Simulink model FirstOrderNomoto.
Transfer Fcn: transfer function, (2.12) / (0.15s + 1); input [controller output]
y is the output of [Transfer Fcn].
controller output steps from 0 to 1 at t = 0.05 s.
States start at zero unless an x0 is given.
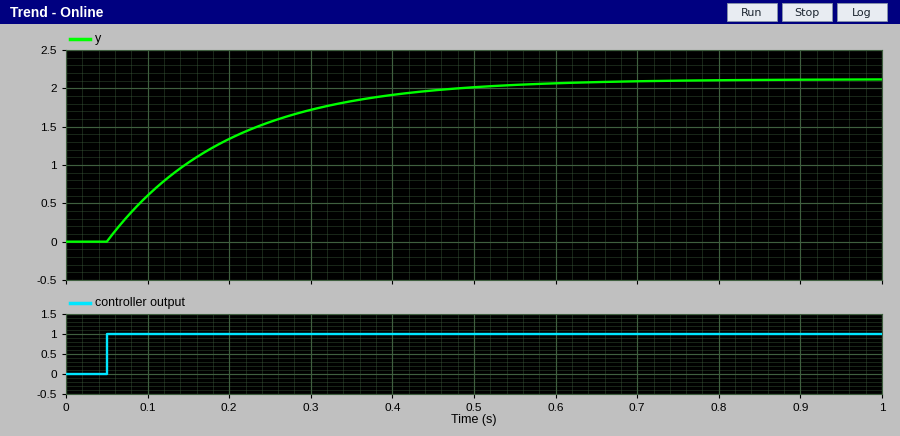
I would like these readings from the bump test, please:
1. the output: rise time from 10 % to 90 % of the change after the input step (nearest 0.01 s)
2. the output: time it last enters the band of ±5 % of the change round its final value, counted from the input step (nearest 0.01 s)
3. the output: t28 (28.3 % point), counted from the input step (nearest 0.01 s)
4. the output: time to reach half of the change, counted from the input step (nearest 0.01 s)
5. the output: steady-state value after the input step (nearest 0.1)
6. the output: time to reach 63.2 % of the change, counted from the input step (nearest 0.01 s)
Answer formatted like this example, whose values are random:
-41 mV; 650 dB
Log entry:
0.33 s; 0.45 s; 0.05 s; 0.10 s; 2.1; 0.15 s
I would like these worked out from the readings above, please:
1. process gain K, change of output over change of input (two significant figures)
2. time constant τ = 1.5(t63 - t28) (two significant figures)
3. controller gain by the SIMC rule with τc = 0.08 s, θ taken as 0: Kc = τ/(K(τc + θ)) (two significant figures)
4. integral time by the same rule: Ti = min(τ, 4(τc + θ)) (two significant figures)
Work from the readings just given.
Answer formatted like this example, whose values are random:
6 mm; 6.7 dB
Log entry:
2.1; 0.15 s; 0.89; 0.15 s
